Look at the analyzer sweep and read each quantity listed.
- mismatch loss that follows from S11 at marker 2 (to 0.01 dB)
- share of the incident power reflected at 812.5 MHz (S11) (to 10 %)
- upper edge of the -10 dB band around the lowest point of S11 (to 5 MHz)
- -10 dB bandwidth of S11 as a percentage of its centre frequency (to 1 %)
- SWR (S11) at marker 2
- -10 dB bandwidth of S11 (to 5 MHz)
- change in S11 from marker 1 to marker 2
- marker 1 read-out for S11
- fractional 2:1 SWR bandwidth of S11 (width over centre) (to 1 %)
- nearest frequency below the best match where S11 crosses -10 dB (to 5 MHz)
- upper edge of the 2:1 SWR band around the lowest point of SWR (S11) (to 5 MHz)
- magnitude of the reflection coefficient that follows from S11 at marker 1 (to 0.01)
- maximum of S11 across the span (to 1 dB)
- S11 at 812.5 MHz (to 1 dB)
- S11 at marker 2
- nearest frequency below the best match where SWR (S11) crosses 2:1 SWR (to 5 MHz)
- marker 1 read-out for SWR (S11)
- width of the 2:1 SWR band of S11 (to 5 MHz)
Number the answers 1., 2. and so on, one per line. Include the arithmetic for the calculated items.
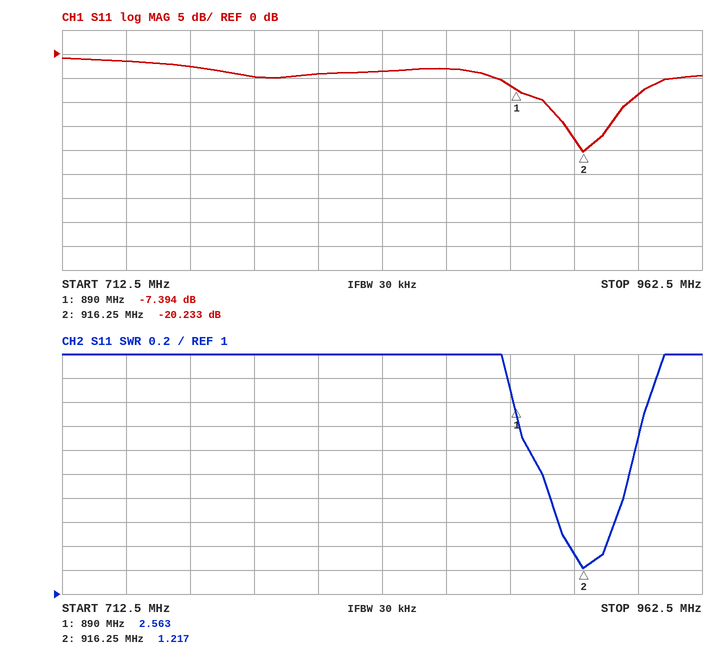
1. −10 log10(1 − 10^(-20.233/10)) ≈ 0.04 dB
2. 10^(-4/10) ≈ 40 %
3. 935 MHz
4. 35 MHz / 917.5 MHz ≈ 4 %
5. 1.217
6. 935 MHz − 900 MHz = 35 MHz
7. -20.233 − (-7.394) = -12.839 dB
8. -7.394 dB
9. 35 MHz / 917.5 MHz ≈ 4 %
10. 900 MHz
11. 935 MHz
12. 10^(-7.394/20) ≈ 0.43
13. -1 dB
14. -4 dB
15. -20.233 dB
16. 900 MHz
17. 2.563
18. 935 MHz − 900 MHz = 35 MHz
